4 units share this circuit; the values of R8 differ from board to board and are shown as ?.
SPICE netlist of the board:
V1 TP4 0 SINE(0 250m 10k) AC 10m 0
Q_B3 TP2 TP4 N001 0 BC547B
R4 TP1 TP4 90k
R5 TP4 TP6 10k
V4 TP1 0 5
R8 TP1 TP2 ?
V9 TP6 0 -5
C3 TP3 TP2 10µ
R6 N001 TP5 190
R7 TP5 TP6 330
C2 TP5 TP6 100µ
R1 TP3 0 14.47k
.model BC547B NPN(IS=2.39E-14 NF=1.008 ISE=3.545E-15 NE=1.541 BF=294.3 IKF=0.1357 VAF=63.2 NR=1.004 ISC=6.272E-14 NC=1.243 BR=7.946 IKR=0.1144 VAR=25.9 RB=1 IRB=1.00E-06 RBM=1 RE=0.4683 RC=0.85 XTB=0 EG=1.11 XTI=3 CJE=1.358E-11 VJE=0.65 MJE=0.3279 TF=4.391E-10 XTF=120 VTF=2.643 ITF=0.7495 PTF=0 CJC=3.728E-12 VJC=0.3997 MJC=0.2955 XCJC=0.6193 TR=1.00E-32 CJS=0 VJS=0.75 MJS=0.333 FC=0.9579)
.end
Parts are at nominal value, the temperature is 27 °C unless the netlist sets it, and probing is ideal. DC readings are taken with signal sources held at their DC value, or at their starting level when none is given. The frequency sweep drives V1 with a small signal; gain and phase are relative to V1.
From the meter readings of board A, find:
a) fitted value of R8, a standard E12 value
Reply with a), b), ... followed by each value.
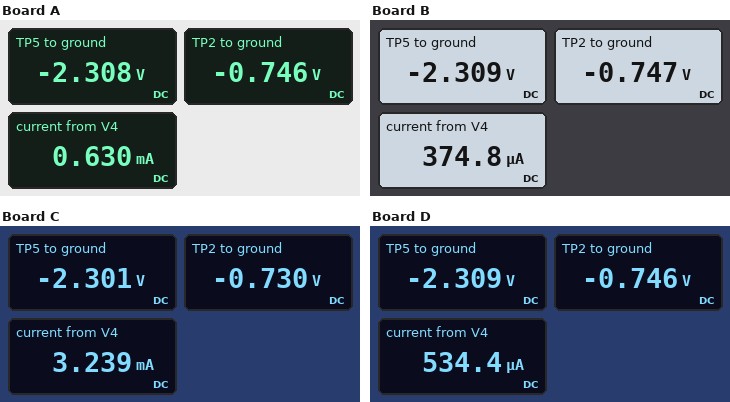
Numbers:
a) 10 kΩ
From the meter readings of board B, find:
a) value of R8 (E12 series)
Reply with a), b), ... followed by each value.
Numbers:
a) 18 kΩ
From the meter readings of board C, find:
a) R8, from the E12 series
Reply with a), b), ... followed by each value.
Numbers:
a) 1.8 kΩ
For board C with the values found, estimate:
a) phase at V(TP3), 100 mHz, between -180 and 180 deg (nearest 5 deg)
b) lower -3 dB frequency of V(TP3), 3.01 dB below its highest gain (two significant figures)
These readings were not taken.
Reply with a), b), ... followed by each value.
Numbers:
a) 85 deg
b) 1.1 Hz
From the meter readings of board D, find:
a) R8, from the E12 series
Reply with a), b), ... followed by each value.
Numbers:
a) 12 kΩ
